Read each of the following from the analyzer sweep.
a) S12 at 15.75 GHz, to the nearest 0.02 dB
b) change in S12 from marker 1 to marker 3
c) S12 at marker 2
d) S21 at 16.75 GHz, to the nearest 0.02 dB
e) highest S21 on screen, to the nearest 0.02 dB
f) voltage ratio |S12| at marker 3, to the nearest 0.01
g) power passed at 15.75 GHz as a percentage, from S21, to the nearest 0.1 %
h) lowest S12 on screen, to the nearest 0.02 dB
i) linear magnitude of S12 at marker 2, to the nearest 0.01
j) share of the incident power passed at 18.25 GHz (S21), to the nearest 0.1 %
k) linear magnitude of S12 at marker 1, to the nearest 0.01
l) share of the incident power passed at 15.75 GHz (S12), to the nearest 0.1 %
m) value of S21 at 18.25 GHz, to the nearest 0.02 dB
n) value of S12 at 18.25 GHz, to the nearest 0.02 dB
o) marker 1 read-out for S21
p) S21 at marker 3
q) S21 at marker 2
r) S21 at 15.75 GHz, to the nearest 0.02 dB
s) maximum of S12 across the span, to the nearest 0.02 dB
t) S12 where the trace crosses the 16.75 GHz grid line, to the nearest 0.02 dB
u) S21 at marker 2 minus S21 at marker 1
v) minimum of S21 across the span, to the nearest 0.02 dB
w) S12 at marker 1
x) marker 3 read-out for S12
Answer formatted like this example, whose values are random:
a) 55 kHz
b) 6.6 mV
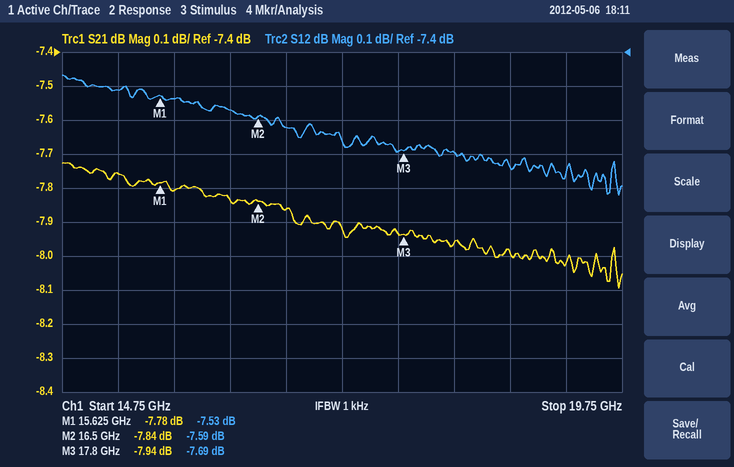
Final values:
a) -7.54 dB
b) -0.16 dB
c) -7.59 dB
d) -7.86 dB
e) -7.72 dB
f) 0.41
g) 16.6 %
h) -7.82 dB
i) 0.42
j) 16.0 %
k) 0.42
l) 17.6 %
m) -7.96 dB
n) -7.70 dB
o) -7.78 dB
p) -7.94 dB
q) -7.84 dB
r) -7.80 dB
s) -7.46 dB
t) -7.62 dB
u) -0.06 dB
v) -8.10 dB
w) -7.53 dB
x) -7.69 dB
